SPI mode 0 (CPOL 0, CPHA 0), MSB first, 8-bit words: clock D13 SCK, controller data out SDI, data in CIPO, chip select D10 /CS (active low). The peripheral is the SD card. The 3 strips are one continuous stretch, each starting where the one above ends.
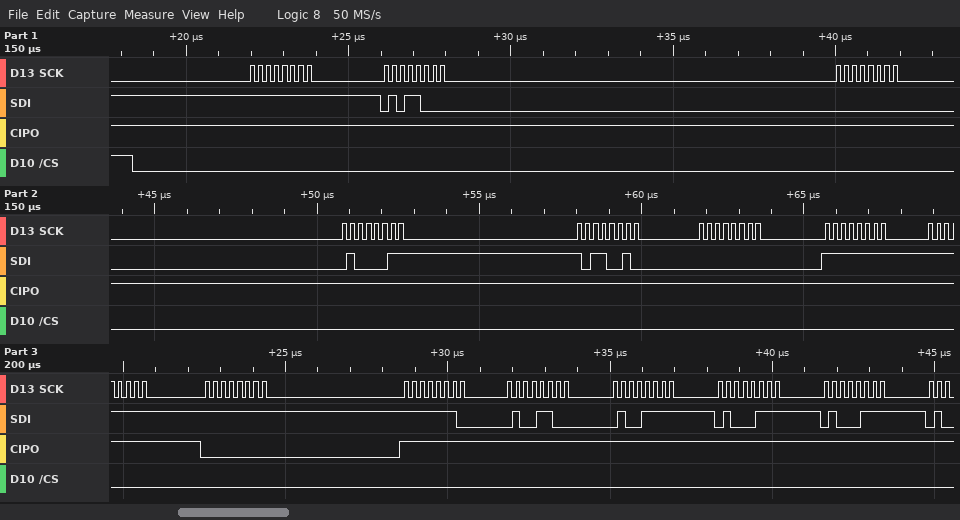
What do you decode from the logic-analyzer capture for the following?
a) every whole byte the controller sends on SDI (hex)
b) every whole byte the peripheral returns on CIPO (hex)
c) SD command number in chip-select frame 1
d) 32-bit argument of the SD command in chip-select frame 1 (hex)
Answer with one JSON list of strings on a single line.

["FF 58 00 43 B2 00 FF FF FF FE 4C 4F 47 47", "FF FF FF FF FF FF FF FF 00 FF FF FF FF FF", "CMD24", "0x0043B200"]
